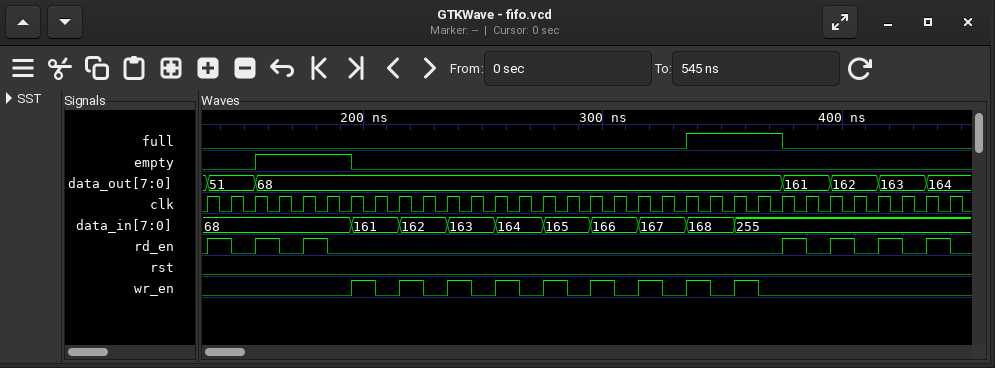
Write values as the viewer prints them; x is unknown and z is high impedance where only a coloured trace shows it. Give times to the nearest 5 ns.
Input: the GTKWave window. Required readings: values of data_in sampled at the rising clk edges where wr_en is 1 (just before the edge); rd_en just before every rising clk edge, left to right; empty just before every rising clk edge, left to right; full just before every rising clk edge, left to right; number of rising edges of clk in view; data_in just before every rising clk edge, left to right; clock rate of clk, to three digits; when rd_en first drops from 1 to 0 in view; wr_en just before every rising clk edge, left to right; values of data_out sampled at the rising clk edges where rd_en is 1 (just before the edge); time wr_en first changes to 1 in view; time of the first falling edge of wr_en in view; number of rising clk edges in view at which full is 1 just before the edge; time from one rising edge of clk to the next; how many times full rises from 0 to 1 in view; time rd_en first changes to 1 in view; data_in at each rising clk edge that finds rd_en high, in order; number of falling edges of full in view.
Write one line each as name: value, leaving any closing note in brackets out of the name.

values of data_in sampled at the rising clk edges where wr_en is 1: 161, 162, 163, 164, 165, 166, 167, 168, 255
rd_en just before every rising clk edge, left to right: 0 1 0 1 0 1 0 0 0 0 0 0 0 0 0 0 0 0 0 0 0 0 0 0 0 1 0 1 0 1 0 1
empty just before every rising clk edge, left to right: 0 0 0 1 1 1 1 0 0 0 0 0 0 0 0 0 0 0 0 0 0 0 0 0 0 0 0 0 0 0 0 0
full just before every rising clk edge, left to right: 0 0 0 0 0 0 0 0 0 0 0 0 0 0 0 0 0 0 0 0 0 1 1 1 1 0 0 0 0 0 0 0
number of rising edges of clk in view: 32
data_in just before every rising clk edge, left to right: 68, 68, 68, 68, 68, 68, 68, 161, 161, 162, 162, 163, 163, 164, 164, 165, 165, 166, 166, 167, 167, 168, 168, 255, 255, 255, 255, 255, 255, 255, 255, 255
clock rate of clk, to three digits: 100 MHz
when rd_en first drops from 1 to 0 in view: 145 ns
wr_en just before every rising clk edge, left to right: 0 0 0 0 0 0 0 1 0 1 0 1 0 1 0 1 0 1 0 1 0 1 0 1 0 0 0 0 0 0 0 0
values of data_out sampled at the rising clk edges where rd_en is 1: 51, 68, 68, 161, 162, 163, 164
time wr_en first changes to 1 in view: 195 ns
time of the first falling edge of wr_en in view: 205 ns
number of rising clk edges in view at which full is 1 just before the edge: 4
time from one rising edge of clk to the next: 10 ns
how many times full rises from 0 to 1 in view: 1
time rd_en first changes to 1 in view: 135 ns
data_in at each rising clk edge that finds rd_en high, in order: 68, 68, 68, 255, 255, 255, 255
number of falling edges of full in view: 1
